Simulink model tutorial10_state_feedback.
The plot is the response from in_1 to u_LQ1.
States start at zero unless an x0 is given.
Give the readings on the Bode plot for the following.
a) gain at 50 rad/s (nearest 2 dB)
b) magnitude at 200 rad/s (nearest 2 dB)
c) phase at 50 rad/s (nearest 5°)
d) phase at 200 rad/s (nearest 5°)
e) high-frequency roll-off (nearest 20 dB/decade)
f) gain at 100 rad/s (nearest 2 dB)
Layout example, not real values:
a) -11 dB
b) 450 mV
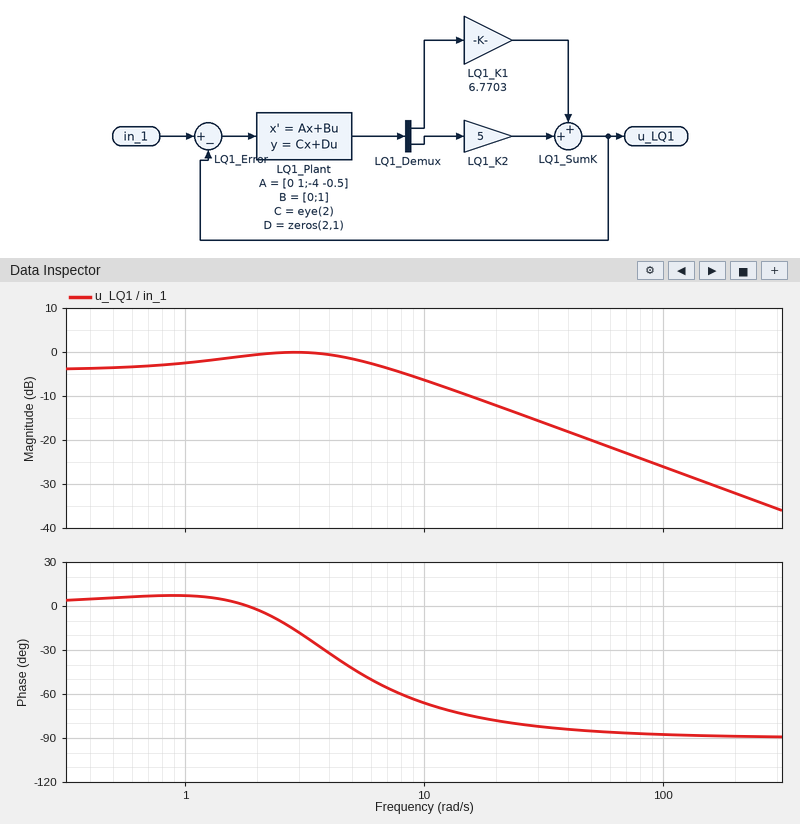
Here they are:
a) -20 dB
b) -32 dB
c) -85°
d) -90°
e) -20 dB/decade
f) -26 dB
